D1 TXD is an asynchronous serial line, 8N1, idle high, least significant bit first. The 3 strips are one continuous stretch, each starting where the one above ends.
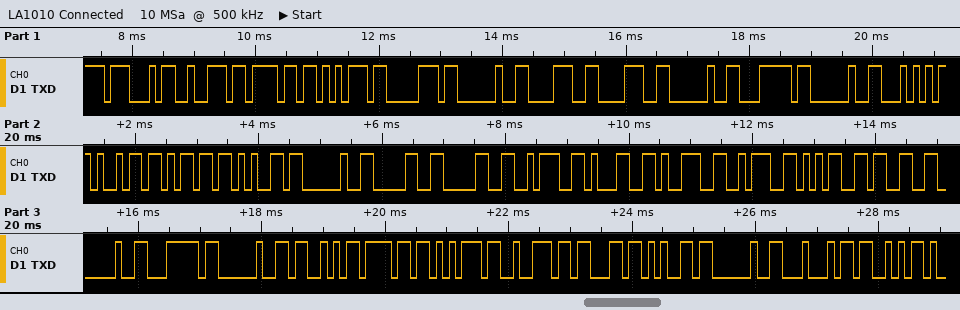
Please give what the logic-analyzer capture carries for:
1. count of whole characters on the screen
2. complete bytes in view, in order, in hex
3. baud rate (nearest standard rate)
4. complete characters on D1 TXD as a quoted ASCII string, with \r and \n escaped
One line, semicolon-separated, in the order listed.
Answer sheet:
36; 0x47 0x72 0x6F 0x75 0x70 0x20 0x38 0x38 0x20 0x7C 0x20 0x54 0x69 0x6D 0x65 0x20 0x30 0x30 0x3A 0x31 0x39 0x3A 0x35 0x33 0x20 0x7C 0x20 0x53 0x6F 0x75 0x72 0x63 0x65 0x20 0x44 0x53; 9600 baud; "Group 88 | Time 00:19:53 | Source DS"
